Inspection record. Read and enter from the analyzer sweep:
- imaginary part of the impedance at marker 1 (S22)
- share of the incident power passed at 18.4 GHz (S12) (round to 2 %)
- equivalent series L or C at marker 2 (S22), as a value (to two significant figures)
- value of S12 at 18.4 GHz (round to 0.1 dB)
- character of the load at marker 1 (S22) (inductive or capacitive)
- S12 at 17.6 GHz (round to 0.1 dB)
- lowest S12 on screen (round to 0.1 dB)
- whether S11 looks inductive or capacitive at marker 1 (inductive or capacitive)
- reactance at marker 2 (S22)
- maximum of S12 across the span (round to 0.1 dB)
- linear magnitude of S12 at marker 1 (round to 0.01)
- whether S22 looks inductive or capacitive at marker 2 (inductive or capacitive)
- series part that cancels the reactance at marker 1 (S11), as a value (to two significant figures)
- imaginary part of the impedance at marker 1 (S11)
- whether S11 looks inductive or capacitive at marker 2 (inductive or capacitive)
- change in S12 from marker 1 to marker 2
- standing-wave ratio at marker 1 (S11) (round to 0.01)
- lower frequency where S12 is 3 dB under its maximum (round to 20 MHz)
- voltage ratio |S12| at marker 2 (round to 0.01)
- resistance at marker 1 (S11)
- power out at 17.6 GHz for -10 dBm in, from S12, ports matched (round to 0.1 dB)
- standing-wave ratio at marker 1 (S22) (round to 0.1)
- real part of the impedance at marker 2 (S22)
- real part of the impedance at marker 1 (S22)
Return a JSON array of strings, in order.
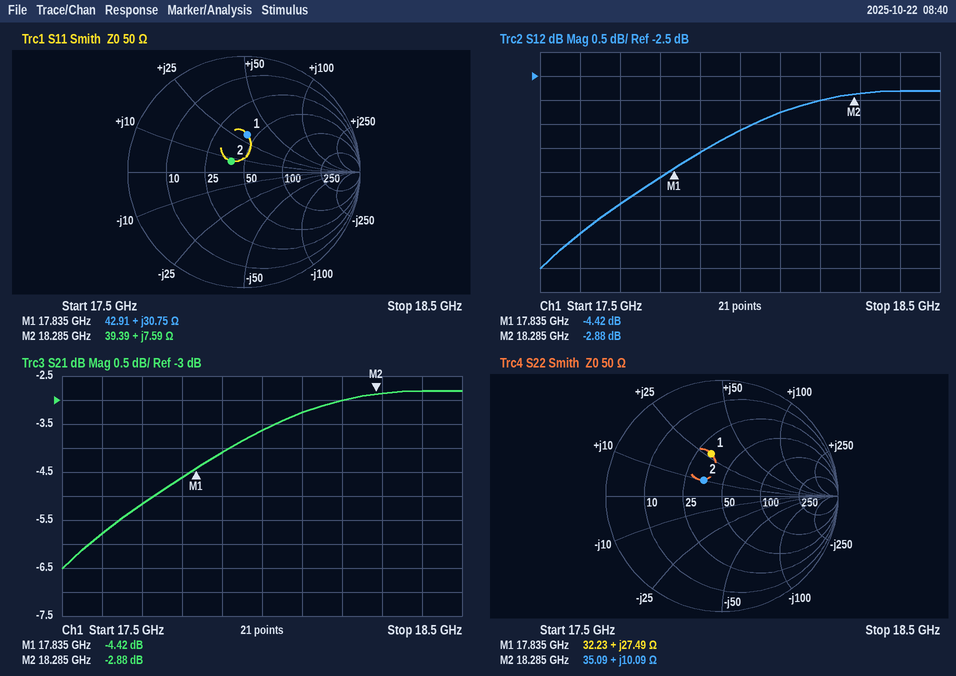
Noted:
["+27.49 Ω", "52 %", "88 pH", "-2.8 dB", "inductive", "-5.8 dB", "-6.5 dB", "inductive", "+10.09 Ω", "-2.8 dB", "0.60", "inductive", "290 fF", "+30.75 Ω", "inductive", "1.54 dB", "1.95", "17.60 GHz", "0.72", "42.91 Ω", "-15.8 dBm", "2.2", "35.09 Ω", "32.23 Ω"]
